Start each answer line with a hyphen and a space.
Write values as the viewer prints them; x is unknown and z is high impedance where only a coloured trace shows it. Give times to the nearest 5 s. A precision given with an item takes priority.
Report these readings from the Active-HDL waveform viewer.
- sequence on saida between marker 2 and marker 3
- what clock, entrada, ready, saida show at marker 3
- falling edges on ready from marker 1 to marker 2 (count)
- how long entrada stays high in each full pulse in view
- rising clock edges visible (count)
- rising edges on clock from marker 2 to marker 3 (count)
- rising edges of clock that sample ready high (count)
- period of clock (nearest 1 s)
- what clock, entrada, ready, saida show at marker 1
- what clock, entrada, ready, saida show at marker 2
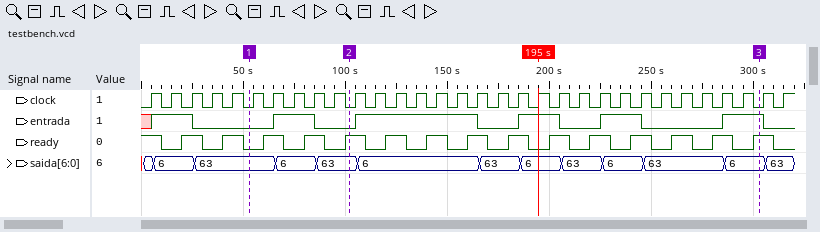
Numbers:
- 63, 6, 63, 6, 63, 6, 63, 6
- clock=0, entrada=1, ready=1, saida=6
- 2
- 20 s, 60 s, 20 s, 20 s, 20 s
- 32
- 20
- 16
- 10 s
- clock=0, entrada=0, ready=0, saida=63
- clock=0, entrada=0, ready=1, saida=63
